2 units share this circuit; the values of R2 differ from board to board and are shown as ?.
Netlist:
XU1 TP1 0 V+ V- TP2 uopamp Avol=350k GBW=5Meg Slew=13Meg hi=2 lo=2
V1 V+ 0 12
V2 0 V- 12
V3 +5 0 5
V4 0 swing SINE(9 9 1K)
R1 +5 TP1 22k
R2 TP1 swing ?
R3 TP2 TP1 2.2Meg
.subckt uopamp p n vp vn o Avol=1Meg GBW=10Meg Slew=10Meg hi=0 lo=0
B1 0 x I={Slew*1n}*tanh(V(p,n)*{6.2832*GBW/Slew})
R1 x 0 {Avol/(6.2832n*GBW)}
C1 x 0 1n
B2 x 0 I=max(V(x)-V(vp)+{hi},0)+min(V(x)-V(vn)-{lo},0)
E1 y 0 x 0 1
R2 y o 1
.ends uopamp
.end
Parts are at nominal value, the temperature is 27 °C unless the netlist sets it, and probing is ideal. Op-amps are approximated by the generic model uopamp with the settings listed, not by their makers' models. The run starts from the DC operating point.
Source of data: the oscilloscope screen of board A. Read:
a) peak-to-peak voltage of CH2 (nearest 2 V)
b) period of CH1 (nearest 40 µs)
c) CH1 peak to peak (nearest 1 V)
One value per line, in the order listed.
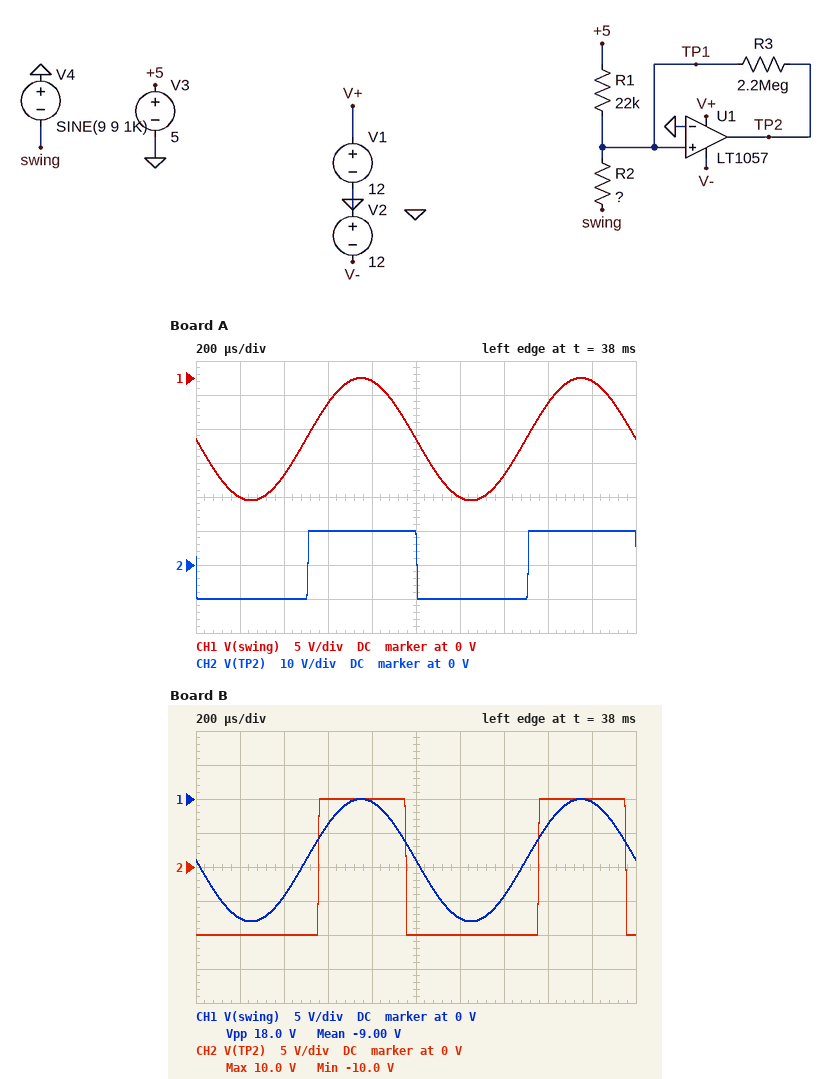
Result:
20 V
1.00 ms
18 V
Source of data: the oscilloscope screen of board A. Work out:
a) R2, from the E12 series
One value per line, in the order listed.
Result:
39 kΩ
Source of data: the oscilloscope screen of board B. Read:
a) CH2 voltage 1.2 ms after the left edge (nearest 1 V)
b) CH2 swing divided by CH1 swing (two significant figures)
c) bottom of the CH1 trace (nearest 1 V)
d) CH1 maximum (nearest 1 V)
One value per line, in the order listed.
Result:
-10 V
1.1
-18 V
0 V
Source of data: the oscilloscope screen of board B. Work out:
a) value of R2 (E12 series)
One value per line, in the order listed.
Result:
27 kΩ
